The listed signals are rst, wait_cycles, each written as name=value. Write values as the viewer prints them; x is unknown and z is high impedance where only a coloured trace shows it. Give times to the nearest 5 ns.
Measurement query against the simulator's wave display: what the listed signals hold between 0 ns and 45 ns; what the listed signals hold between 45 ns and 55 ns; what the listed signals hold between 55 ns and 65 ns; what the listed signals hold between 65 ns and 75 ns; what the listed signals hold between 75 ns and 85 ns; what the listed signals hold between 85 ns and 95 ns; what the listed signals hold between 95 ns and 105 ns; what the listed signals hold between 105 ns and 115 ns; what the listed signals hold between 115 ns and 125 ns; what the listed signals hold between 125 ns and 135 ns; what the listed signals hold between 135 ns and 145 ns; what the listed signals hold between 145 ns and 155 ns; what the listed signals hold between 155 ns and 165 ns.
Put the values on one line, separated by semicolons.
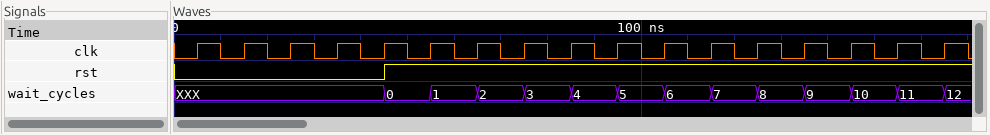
rst=0, wait_cycles=XXX; rst=1, wait_cycles=0; rst=1, wait_cycles=1; rst=1, wait_cycles=2; rst=1, wait_cycles=3; rst=1, wait_cycles=4; rst=1, wait_cycles=5; rst=1, wait_cycles=6; rst=1, wait_cycles=7; rst=1, wait_cycles=8; rst=1, wait_cycles=9; rst=1, wait_cycles=10; rst=1, wait_cycles=11
